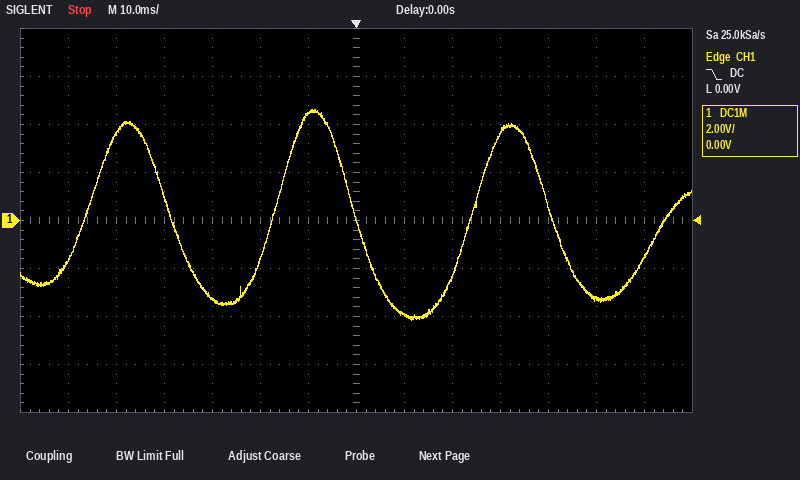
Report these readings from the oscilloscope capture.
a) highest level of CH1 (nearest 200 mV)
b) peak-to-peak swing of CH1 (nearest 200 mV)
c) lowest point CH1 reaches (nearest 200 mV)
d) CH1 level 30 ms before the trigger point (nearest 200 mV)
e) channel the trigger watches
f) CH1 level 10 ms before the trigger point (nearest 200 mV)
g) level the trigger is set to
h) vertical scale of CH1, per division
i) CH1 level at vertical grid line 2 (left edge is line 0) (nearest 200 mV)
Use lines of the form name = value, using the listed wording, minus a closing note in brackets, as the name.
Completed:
highest level of CH1 = 4.6 V
peak-to-peak swing of CH1 = 8.8 V
lowest point CH1 reaches = -4.2 V
CH1 level 30 ms before the trigger point = -3.2 V
channel the trigger watches = CH1
CH1 level 10 ms before the trigger point = 4.4 V
level the trigger is set to = 0.00 V
vertical scale of CH1, per division = 2 V
CH1 level at vertical grid line 2 (left edge is line 0) = 3.6 V
